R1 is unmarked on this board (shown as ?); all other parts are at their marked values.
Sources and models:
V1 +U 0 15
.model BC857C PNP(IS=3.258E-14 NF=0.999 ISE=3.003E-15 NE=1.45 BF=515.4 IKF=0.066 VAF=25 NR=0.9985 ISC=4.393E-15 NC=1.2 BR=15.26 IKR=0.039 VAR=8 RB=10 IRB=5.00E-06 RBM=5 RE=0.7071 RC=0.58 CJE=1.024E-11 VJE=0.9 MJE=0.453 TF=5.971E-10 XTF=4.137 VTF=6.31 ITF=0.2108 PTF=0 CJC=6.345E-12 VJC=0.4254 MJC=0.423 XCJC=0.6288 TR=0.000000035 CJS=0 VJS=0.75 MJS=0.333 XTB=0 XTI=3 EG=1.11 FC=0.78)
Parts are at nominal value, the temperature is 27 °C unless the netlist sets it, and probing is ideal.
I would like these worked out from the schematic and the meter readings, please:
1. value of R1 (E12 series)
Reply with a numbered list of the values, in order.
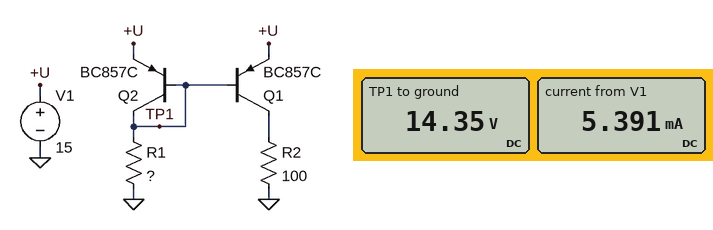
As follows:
1. 6.8 kΩ
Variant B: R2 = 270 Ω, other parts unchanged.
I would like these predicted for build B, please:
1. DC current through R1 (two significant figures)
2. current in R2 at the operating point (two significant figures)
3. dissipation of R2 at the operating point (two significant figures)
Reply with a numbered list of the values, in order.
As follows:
1. 2.1 mA
2. 3.2 mA
3. 2.8 mW
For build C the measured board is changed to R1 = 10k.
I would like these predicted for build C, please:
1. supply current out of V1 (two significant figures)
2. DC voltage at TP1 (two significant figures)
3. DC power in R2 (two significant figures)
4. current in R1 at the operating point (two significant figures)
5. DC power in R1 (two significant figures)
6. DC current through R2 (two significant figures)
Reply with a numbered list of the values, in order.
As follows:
1. 3.7 mA
2. 14 V
3. 510 µW
4. 1.4 mA
5. 21 mW
6. 2.3 mA
